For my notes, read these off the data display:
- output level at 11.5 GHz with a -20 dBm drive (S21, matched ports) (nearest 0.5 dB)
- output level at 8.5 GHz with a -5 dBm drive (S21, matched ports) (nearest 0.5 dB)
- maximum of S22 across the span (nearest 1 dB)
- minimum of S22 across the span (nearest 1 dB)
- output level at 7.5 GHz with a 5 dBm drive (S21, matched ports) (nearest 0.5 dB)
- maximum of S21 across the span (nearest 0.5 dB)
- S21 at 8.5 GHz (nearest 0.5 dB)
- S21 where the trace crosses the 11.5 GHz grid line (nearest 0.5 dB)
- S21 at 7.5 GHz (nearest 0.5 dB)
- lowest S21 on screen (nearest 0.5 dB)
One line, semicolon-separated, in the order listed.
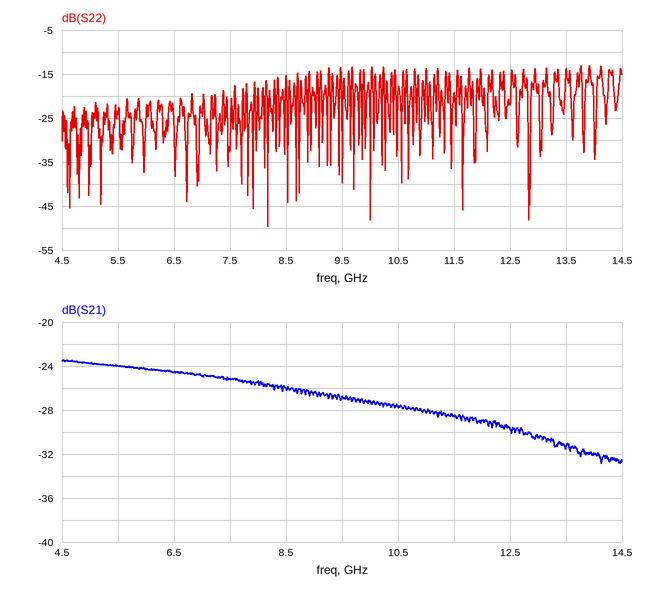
-48.5 dBm; -31.0 dBm; -13 dB; -50 dB; -20.0 dBm; -23.5 dB; -26.0 dB; -28.5 dB; -25.0 dB; -33.0 dB
